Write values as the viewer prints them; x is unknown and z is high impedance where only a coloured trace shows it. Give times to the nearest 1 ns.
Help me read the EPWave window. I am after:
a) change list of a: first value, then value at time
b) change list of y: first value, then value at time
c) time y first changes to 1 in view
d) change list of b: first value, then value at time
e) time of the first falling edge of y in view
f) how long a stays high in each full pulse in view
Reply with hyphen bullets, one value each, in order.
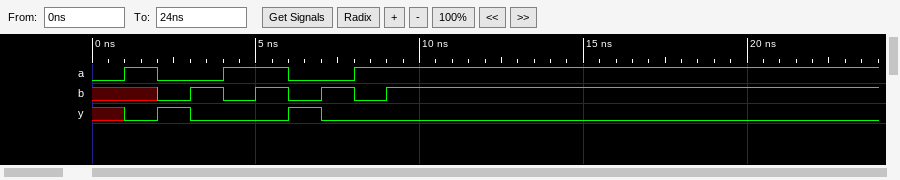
- 0, 1 at 1 ns, 0 at 2 ns, 1 at 4 ns, 0 at 6 ns, 1 at 8 ns
- x, 0 at 1 ns, 1 at 2 ns, 0 at 3 ns, 1 at 6 ns, 0 at 7 ns
- 2 ns
- x, 0 at 2 ns, 1 at 3 ns, 0 at 4 ns, 1 at 5 ns, 0 at 6 ns, 1 at 7 ns, 0 at 8 ns, 1 at 9 ns
- 3 ns
- 1 ns, 2 ns
